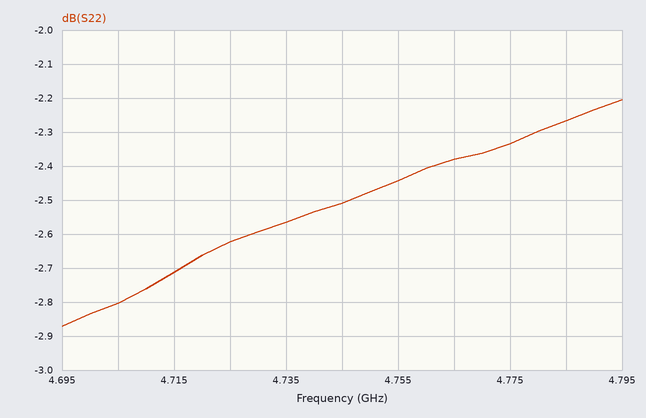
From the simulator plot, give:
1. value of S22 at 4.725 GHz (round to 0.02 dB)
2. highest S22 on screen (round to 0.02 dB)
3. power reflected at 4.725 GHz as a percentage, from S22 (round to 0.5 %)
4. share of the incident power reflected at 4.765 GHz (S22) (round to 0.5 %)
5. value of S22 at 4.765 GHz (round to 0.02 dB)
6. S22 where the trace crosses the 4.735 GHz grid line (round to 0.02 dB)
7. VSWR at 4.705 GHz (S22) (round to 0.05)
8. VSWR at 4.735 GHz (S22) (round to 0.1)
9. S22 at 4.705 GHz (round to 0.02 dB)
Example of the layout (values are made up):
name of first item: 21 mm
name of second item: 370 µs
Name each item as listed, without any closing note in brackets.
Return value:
value of S22 at 4.725 GHz: -2.62 dB
highest S22 on screen: -2.20 dB
power reflected at 4.725 GHz as a percentage, from S22: 54.5 %
share of the incident power reflected at 4.765 GHz (S22): 58.0 %
value of S22 at 4.765 GHz: -2.38 dB
S22 where the trace crosses the 4.735 GHz grid line: -2.56 dB
VSWR at 4.705 GHz (S22): 6.25
VSWR at 4.735 GHz (S22): 6.8
S22 at 4.705 GHz: -2.80 dB
